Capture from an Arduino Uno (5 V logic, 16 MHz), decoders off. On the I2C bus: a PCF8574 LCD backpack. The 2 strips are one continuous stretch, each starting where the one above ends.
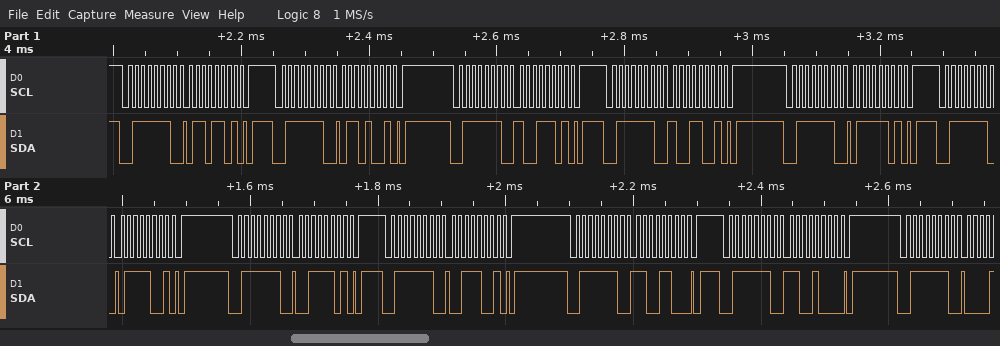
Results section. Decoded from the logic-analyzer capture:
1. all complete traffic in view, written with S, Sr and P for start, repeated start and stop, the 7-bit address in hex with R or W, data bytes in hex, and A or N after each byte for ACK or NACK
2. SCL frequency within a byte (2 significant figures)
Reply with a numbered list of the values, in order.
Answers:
1. S 3FW A 6D A P S 3FW A 69 A P S 3FW A 9D A P S 3FW A 99 A P S 3FW A 7D A P S 3FW A 79 A P S 3FW A 3D A P S 3FW A 39 A P S 3FW A CC A P S 3FW A C8 A P S 3FW A
2. 100 kHz
